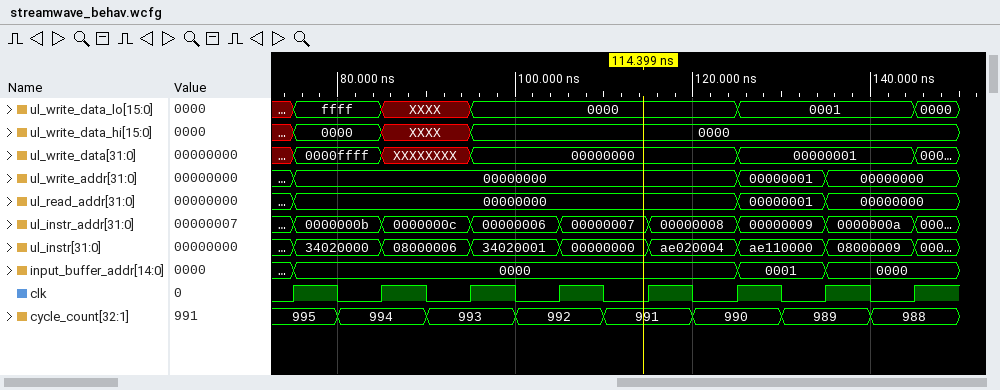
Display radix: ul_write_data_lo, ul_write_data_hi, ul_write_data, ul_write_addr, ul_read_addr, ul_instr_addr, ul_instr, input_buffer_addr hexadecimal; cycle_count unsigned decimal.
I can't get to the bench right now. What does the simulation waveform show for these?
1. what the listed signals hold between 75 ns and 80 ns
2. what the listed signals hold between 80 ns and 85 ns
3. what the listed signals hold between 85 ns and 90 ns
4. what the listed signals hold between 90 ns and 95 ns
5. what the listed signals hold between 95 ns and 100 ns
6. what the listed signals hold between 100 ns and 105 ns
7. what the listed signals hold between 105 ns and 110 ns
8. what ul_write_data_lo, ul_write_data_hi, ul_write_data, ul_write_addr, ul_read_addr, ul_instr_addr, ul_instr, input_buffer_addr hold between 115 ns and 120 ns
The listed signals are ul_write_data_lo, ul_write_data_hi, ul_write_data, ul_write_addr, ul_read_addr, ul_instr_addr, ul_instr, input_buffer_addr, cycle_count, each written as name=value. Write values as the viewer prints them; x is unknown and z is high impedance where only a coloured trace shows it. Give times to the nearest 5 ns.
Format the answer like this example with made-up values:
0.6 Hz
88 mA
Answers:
ul_write_data_lo=ffff, ul_write_data_hi=0000, ul_write_data=0000ffff, ul_write_addr=00000000, ul_read_addr=00000000, ul_instr_addr=0000000b, ul_instr=34020000, input_buffer_addr=0000, cycle_count=995
ul_write_data_lo=ffff, ul_write_data_hi=0000, ul_write_data=0000ffff, ul_write_addr=00000000, ul_read_addr=00000000, ul_instr_addr=0000000b, ul_instr=34020000, input_buffer_addr=0000, cycle_count=994
ul_write_data_lo=XXXX, ul_write_data_hi=XXXX, ul_write_data=XXXXXXXX, ul_write_addr=00000000, ul_read_addr=00000000, ul_instr_addr=0000000c, ul_instr=08000006, input_buffer_addr=0000, cycle_count=994
ul_write_data_lo=XXXX, ul_write_data_hi=XXXX, ul_write_data=XXXXXXXX, ul_write_addr=00000000, ul_read_addr=00000000, ul_instr_addr=0000000c, ul_instr=08000006, input_buffer_addr=0000, cycle_count=993
ul_write_data_lo=0000, ul_write_data_hi=0000, ul_write_data=00000000, ul_write_addr=00000000, ul_read_addr=00000000, ul_instr_addr=00000006, ul_instr=34020001, input_buffer_addr=0000, cycle_count=993
ul_write_data_lo=0000, ul_write_data_hi=0000, ul_write_data=00000000, ul_write_addr=00000000, ul_read_addr=00000000, ul_instr_addr=00000006, ul_instr=34020001, input_buffer_addr=0000, cycle_count=992
ul_write_data_lo=0000, ul_write_data_hi=0000, ul_write_data=00000000, ul_write_addr=00000000, ul_read_addr=00000000, ul_instr_addr=00000007, ul_instr=00000000, input_buffer_addr=0000, cycle_count=992
ul_write_data_lo=0000, ul_write_data_hi=0000, ul_write_data=00000000, ul_write_addr=00000000, ul_read_addr=00000000, ul_instr_addr=00000008, ul_instr=ae020004, input_buffer_addr=0000
